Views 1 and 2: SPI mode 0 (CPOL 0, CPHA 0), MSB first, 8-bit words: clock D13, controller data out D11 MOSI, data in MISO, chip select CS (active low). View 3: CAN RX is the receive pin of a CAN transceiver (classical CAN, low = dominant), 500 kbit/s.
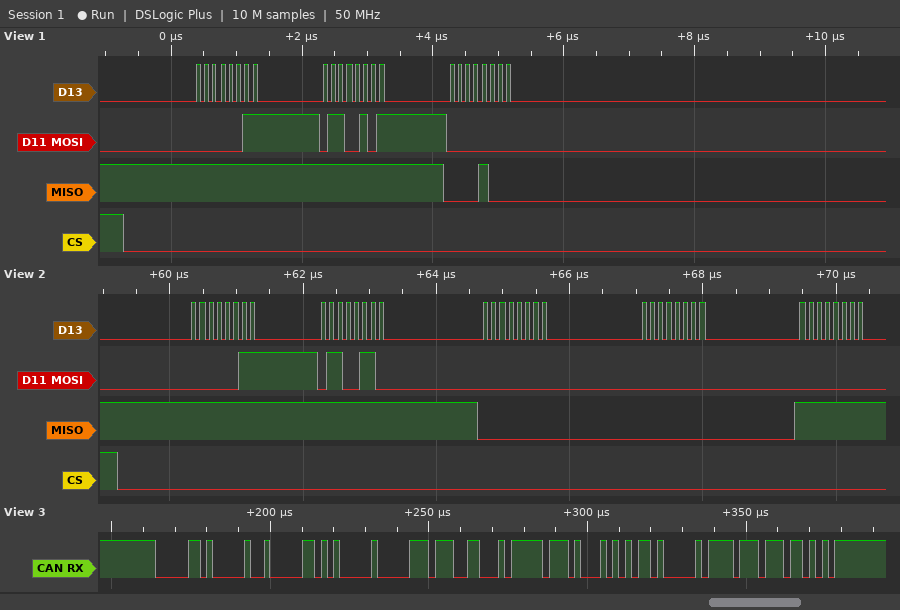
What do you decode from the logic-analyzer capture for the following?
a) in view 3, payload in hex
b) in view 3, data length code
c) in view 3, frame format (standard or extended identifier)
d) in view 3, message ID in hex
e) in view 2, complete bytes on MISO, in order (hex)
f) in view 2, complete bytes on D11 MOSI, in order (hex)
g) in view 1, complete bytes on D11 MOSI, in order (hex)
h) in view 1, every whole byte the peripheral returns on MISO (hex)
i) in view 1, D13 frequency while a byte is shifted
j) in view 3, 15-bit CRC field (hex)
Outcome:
2A 00 6E 62 FF 45 5A 07
8
standard
0x050
0xFF 0xFF 0x00 0x00 0xFF
0x03 0x66 0x00 0x00 0x00
03 65 00
FF FF 08
8 MHz
0x5DDA
